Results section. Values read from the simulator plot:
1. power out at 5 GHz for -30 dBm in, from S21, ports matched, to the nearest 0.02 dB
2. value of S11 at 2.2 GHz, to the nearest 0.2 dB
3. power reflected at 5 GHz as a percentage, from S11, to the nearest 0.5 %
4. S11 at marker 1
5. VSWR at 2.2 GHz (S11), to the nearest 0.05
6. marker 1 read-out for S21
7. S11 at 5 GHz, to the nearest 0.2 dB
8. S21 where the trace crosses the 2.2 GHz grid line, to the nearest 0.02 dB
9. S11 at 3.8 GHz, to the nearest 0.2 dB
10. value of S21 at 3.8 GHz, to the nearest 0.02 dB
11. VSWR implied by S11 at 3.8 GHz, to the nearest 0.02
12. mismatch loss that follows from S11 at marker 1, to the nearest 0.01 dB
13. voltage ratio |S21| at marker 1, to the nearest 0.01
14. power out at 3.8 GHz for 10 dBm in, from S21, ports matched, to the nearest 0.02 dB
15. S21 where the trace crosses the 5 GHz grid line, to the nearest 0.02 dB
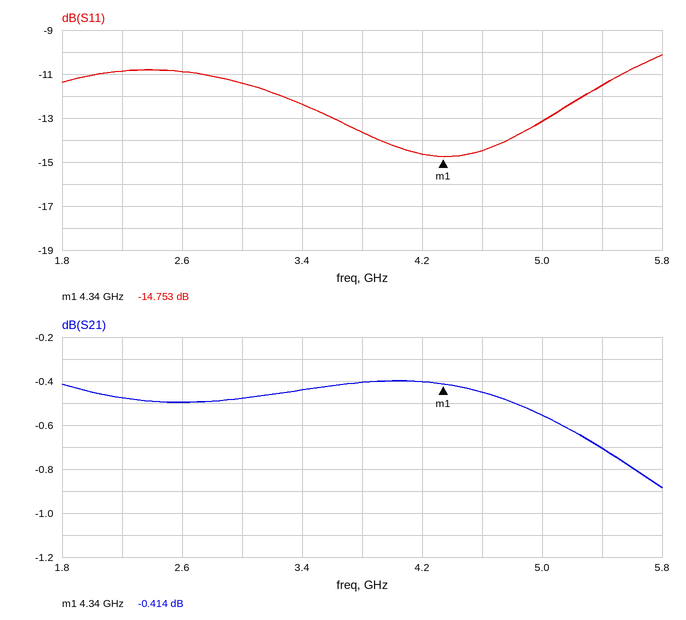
-30.56 dBm
-10.8 dB
5.0 %
-14.753 dB
1.80
-0.414 dB
-13.2 dB
-0.48 dB
-13.6 dB
-0.40 dB
1.52
0.15 dB
0.95
9.60 dBm
-0.56 dB
